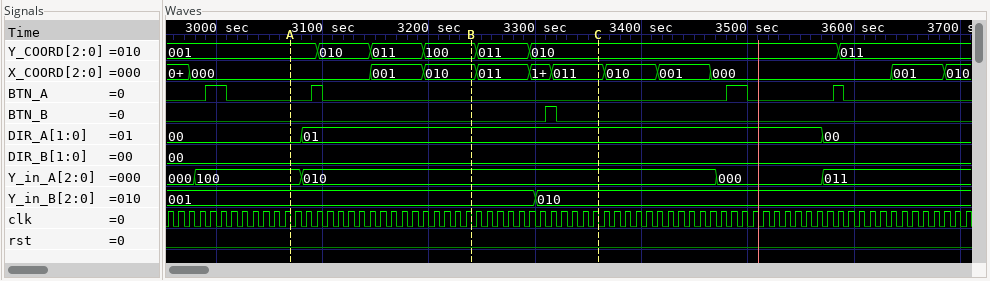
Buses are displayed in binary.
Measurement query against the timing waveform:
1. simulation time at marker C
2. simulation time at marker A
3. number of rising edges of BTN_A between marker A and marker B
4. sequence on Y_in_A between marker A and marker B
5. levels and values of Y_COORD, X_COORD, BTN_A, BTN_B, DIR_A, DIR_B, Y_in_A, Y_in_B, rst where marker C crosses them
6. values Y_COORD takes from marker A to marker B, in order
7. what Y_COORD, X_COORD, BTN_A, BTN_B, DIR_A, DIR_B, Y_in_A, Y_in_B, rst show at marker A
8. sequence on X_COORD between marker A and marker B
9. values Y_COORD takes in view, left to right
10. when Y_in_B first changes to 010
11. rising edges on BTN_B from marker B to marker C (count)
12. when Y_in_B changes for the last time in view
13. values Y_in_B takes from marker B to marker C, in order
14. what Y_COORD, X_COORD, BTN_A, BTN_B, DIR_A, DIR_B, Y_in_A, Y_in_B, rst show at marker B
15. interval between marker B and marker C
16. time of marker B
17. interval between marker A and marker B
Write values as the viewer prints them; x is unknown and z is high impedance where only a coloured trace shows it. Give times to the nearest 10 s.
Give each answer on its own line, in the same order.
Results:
3360 s
3070 s
1
100, 010
Y_COORD=010, X_COORD=011, BTN_A=0, BTN_B=0, DIR_A=01, DIR_B=00, Y_in_A=010, Y_in_B=010, rst=0
001, 010, 011, 100
Y_COORD=001, X_COORD=000, BTN_A=0, BTN_B=0, DIR_A=00, DIR_B=00, Y_in_A=100, Y_in_B=001, rst=0
000, 001, 010
001, 010, 011, 100, 011, 010, 011
3300 s
1
3300 s
001, 010
Y_COORD=100, X_COORD=010, BTN_A=0, BTN_B=0, DIR_A=01, DIR_B=00, Y_in_A=010, Y_in_B=001, rst=0
120 s
3240 s
170 s
